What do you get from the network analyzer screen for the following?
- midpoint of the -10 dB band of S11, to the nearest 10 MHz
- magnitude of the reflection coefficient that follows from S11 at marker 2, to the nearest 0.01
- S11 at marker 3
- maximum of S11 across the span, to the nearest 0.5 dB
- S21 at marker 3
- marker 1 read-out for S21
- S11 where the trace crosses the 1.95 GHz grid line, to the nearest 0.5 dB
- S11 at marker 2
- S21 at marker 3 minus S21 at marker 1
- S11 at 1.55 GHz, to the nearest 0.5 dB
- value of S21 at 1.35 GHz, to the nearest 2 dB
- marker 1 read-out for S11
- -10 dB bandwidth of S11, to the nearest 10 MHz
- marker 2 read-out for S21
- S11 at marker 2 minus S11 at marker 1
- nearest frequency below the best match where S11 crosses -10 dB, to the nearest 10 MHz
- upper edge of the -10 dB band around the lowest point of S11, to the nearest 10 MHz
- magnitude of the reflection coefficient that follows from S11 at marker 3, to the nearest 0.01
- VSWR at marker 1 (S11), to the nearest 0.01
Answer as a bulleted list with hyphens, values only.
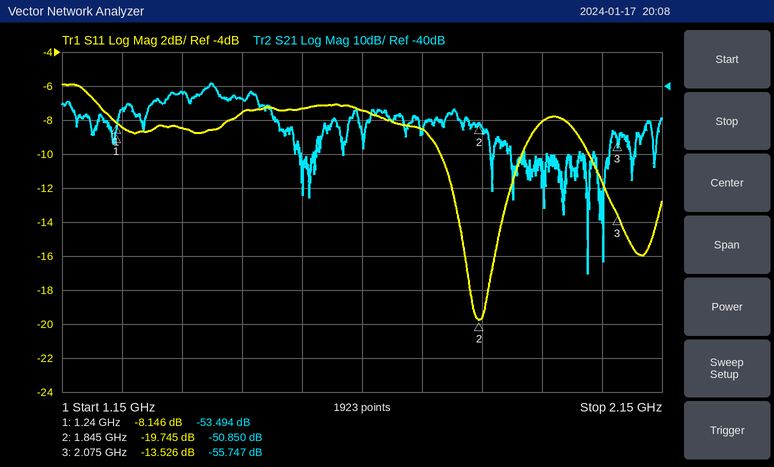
- 1.85 GHz
- 0.10
- -13.526 dB
- -6.0 dB
- -55.747 dB
- -53.494 dB
- -8.0 dB
- -19.745 dB
- -2.253 dB
- -7.5 dB
- -42 dB
- -8.146 dB
- 140 MHz
- -50.850 dB
- -11.599 dB
- 1.78 GHz
- 1.92 GHz
- 0.21
- 2.29
